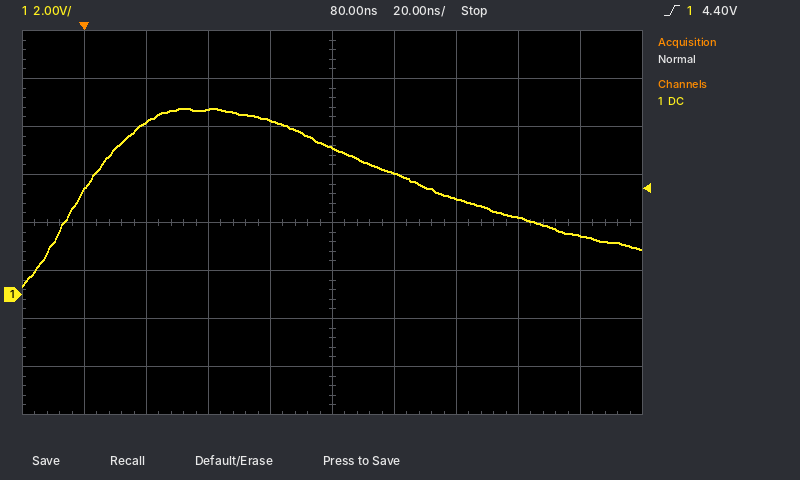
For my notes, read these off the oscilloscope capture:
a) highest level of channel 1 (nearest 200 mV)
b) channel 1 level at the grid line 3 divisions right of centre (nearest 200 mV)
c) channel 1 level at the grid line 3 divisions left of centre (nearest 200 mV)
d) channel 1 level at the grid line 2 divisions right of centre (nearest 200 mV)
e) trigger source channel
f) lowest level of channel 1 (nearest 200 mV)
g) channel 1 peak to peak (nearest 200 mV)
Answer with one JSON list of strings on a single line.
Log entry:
["7.8 V", "3.2 V", "7.2 V", "4.0 V", "channel 1", "400 mV", "7.4 V"]
